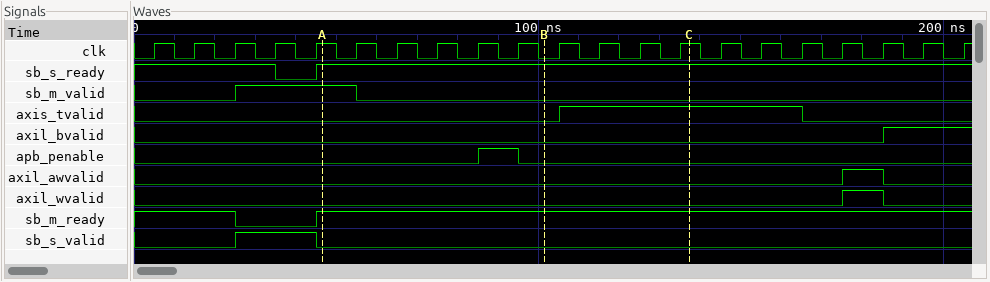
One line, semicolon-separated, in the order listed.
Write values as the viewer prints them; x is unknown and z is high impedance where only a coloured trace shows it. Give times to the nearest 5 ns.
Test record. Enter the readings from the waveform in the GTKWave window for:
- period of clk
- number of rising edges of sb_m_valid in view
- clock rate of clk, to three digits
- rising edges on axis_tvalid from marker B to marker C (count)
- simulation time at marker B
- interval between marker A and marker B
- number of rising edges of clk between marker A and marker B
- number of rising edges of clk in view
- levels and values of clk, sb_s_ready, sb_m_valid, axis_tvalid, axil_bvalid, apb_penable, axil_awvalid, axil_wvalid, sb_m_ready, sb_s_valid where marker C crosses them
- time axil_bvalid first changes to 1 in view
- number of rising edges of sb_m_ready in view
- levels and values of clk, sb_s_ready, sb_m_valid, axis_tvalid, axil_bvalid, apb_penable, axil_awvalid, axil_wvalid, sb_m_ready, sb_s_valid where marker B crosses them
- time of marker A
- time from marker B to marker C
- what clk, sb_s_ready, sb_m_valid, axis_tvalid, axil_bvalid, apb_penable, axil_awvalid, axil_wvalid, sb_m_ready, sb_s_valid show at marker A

10 ns; 1; 100 MHz; 1; 100 ns; 55 ns; 5; 21; clk=1, sb_s_ready=1, sb_m_valid=0, axis_tvalid=1, axil_bvalid=0, apb_penable=0, axil_awvalid=0, axil_wvalid=0, sb_m_ready=1, sb_s_valid=0; 185 ns; 1; clk=0, sb_s_ready=1, sb_m_valid=0, axis_tvalid=0, axil_bvalid=0, apb_penable=0, axil_awvalid=0, axil_wvalid=0, sb_m_ready=1, sb_s_valid=0; 45 ns; 35 ns; clk=1, sb_s_ready=1, sb_m_valid=1, axis_tvalid=0, axil_bvalid=0, apb_penable=0, axil_awvalid=0, axil_wvalid=0, sb_m_ready=1, sb_s_valid=0
